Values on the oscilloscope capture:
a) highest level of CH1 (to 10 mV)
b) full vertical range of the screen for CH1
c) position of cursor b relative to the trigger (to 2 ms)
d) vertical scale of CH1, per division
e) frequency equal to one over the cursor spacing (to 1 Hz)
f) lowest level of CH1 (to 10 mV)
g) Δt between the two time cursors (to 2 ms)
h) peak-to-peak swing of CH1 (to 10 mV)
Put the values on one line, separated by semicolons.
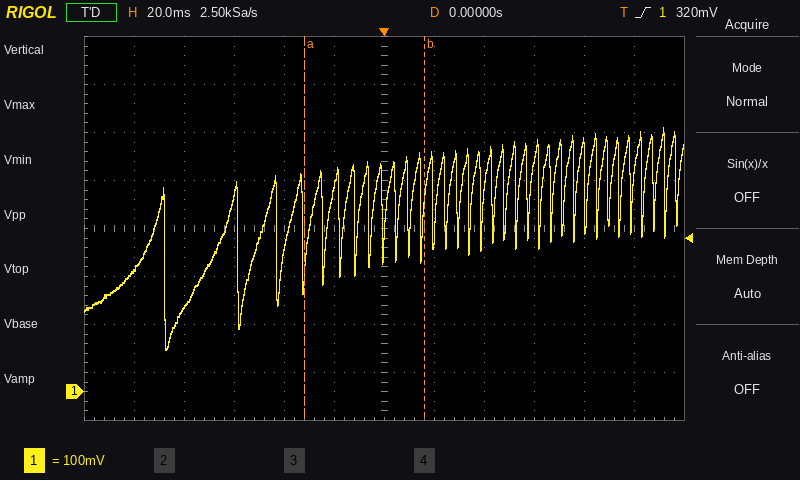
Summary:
550 mV; 800 mV; +16 ms; 100 mV; 21 Hz; 90 mV; 48 ms; 460 mV
